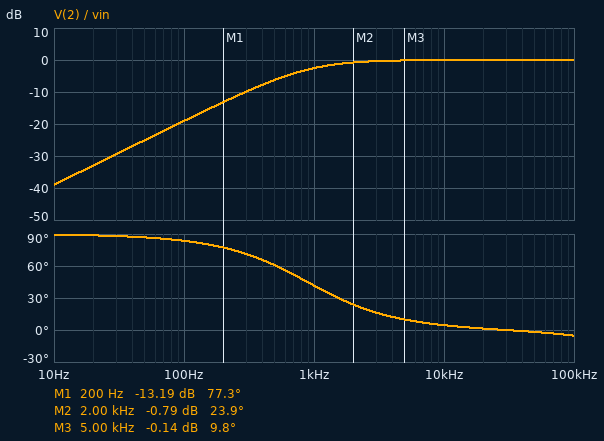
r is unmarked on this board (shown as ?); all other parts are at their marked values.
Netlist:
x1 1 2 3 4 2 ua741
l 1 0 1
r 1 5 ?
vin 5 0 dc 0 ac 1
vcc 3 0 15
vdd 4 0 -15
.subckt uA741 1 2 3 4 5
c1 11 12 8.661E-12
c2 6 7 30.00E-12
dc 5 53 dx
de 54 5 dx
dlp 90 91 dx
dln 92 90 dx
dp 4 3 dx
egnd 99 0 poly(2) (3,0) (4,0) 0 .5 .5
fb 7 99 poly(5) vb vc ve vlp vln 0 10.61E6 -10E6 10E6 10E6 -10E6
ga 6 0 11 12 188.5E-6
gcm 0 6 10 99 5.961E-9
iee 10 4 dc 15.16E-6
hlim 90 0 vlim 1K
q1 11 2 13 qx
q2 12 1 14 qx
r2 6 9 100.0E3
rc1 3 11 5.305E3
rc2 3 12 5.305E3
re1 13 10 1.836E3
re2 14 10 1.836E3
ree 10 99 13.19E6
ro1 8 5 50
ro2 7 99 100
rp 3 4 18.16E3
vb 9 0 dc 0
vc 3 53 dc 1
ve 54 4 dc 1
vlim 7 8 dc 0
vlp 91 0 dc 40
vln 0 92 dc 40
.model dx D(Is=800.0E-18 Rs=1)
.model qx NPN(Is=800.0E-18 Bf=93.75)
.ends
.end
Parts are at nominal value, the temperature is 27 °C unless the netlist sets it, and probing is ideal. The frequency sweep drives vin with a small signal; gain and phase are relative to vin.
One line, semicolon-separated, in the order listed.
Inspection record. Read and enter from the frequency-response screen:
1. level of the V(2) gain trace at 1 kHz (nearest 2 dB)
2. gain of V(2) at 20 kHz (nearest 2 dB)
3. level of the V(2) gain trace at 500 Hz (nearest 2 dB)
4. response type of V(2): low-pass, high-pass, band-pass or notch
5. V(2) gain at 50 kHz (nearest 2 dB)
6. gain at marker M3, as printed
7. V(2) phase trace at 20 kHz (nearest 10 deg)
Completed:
-2 dB; 0 dB; -6 dB; high-pass; 0 dB; -0.14 dB; 0 deg
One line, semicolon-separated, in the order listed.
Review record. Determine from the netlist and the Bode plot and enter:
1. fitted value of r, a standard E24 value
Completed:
5.6 kΩ
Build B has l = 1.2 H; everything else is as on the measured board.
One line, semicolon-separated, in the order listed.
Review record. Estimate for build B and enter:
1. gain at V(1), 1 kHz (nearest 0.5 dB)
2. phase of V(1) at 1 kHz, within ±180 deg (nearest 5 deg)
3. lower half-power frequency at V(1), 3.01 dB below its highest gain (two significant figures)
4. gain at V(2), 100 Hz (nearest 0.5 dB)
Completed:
-2.0 dB; 35 deg; 740 Hz; -17.5 dB
